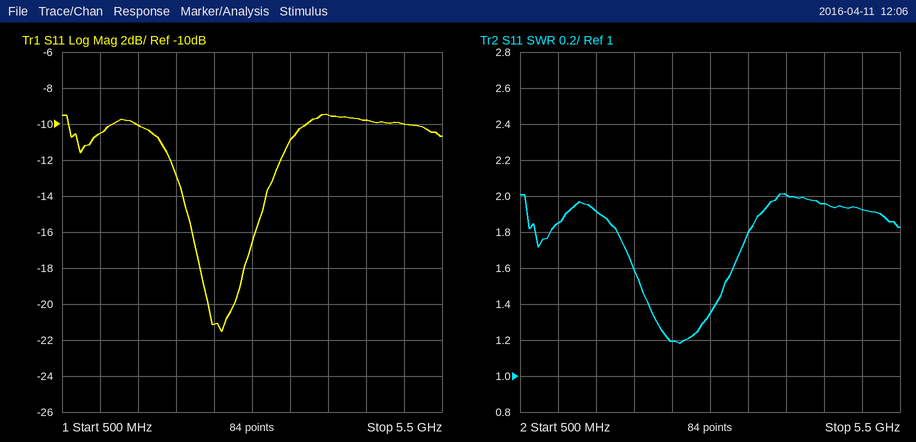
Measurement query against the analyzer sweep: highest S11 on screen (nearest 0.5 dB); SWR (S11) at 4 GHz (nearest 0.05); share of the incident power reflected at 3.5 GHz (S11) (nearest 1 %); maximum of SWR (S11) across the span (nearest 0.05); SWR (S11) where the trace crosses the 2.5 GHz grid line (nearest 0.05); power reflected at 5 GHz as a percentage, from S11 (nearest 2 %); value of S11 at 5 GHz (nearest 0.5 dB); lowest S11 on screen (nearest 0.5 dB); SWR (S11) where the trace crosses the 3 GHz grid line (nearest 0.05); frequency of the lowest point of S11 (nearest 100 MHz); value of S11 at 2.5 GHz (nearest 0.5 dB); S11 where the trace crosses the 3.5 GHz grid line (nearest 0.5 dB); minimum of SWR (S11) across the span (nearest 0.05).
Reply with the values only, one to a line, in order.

-9.5 dB
2.00
8 %
2.00
1.20
10 %
-10.0 dB
-21.5 dB
1.35
2.6 GHz
-21.0 dB
-11.0 dB
1.20
